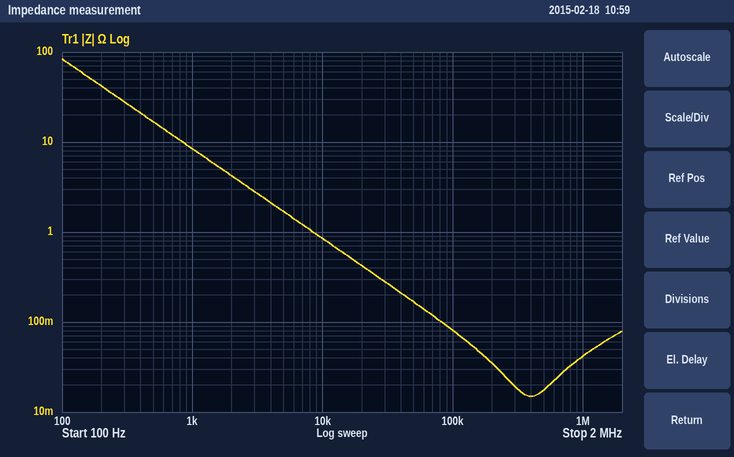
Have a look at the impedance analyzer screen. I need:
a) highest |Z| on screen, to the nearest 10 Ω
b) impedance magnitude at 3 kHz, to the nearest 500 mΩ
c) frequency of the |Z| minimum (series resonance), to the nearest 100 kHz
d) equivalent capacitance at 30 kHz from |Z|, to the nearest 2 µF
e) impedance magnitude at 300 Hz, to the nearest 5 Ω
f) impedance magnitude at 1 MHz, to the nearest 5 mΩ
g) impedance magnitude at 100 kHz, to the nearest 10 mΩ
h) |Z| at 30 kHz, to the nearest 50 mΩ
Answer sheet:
80 Ω
3.0 Ω
400 kHz
18 µF
30 Ω
40 mΩ
80 mΩ
300 mΩ
